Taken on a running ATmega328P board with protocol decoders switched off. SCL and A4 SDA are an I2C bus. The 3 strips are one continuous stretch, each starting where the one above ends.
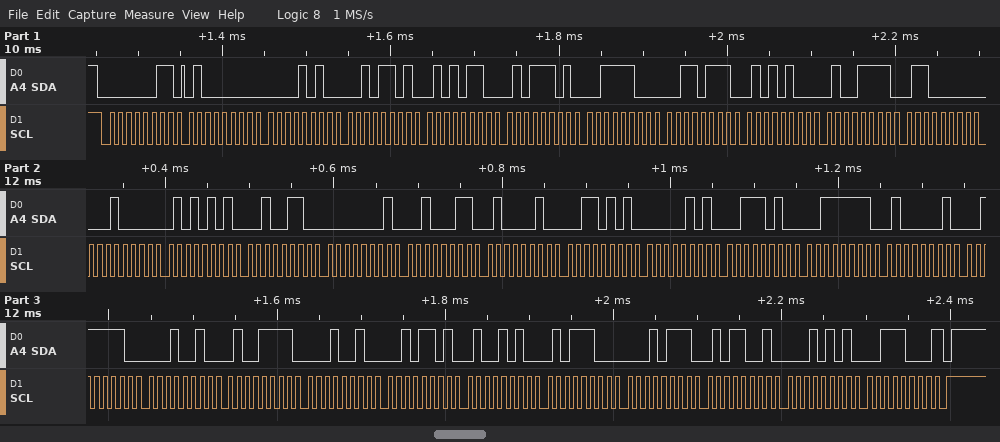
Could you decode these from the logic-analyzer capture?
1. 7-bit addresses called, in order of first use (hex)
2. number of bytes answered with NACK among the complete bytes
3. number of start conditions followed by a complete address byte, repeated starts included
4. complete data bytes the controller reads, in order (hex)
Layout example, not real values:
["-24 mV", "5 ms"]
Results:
["0x01", "1", "1", "40 0A 2D 56 5D 3C 37 54 4F 60 10 55 26 01 23 42 35 05 3A 3F 41 3E 12 4F 12 2D 4A 5C 17 59 15 38"]
